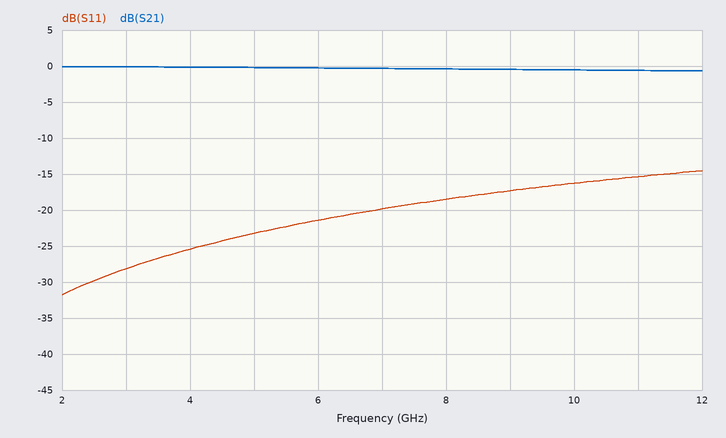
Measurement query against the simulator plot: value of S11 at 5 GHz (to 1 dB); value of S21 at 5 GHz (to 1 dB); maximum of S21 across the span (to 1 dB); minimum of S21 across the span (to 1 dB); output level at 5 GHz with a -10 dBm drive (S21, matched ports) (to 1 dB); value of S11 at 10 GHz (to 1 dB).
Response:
-23 dB
0 dB
0 dB
-1 dB
-10 dBm
-16 dB
